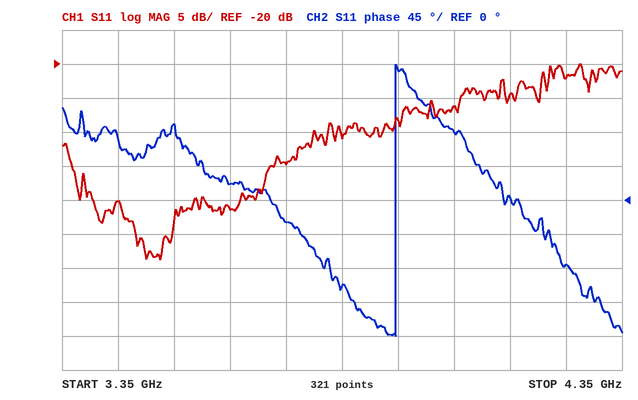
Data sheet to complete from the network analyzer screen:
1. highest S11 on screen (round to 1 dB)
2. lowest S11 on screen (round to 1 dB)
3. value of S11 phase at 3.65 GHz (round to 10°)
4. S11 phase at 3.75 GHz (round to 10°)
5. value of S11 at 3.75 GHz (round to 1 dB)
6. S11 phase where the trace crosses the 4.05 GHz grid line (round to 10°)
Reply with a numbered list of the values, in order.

1. -20 dB
2. -49 dB
3. 20°
4. -30°
5. -35 dB
6. 90°
